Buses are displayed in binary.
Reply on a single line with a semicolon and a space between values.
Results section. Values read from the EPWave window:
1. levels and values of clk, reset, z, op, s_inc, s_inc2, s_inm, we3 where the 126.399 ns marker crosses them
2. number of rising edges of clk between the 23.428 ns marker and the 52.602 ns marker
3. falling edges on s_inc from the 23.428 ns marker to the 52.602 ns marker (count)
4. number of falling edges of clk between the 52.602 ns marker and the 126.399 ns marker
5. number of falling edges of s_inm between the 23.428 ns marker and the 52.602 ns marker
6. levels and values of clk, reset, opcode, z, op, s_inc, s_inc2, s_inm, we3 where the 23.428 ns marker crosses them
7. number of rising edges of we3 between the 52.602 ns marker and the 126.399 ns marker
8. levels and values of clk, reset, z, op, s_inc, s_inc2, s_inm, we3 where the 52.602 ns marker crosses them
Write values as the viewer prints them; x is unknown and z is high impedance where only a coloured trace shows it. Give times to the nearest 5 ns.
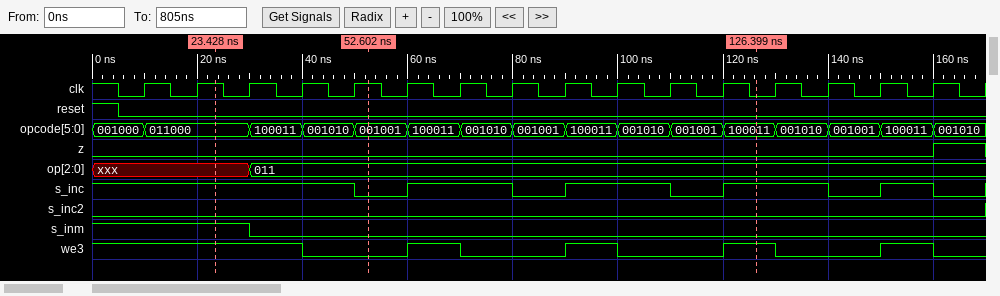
clk=0, reset=0, z=0, op=011, s_inc=1, s_inc2=0, s_inm=0, we3=1; 3; 1; 8; 1; clk=1, reset=0, opcode=011000, z=0, op=xxx, s_inc=1, s_inc2=0, s_inm=1, we3=1; 3; clk=1, reset=0, z=0, op=011, s_inc=0, s_inc2=0, s_inm=0, we3=0
